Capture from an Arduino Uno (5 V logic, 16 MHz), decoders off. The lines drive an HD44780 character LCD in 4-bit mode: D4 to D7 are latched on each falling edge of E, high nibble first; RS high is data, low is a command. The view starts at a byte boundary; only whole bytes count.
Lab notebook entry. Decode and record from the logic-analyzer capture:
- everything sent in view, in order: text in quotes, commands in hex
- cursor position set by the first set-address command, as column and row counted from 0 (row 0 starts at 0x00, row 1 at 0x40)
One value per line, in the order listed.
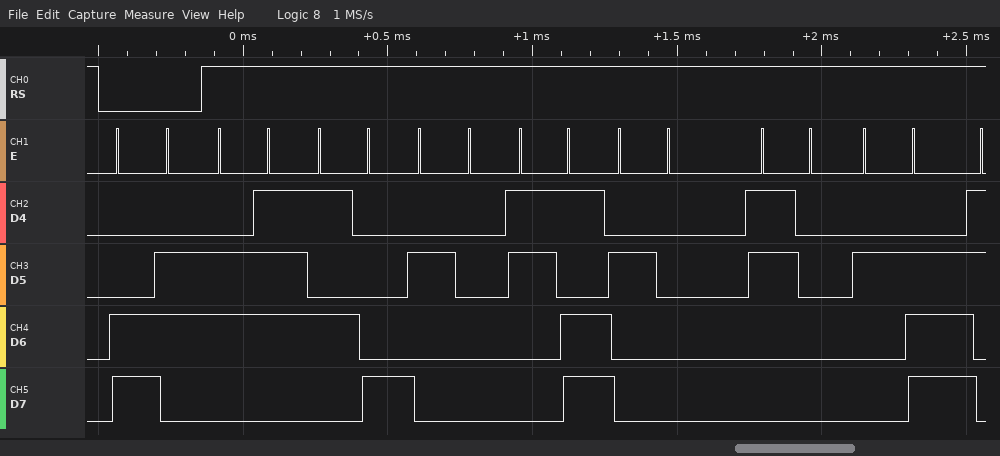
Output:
0xC6 "gX = 0."
column 6, row 1
